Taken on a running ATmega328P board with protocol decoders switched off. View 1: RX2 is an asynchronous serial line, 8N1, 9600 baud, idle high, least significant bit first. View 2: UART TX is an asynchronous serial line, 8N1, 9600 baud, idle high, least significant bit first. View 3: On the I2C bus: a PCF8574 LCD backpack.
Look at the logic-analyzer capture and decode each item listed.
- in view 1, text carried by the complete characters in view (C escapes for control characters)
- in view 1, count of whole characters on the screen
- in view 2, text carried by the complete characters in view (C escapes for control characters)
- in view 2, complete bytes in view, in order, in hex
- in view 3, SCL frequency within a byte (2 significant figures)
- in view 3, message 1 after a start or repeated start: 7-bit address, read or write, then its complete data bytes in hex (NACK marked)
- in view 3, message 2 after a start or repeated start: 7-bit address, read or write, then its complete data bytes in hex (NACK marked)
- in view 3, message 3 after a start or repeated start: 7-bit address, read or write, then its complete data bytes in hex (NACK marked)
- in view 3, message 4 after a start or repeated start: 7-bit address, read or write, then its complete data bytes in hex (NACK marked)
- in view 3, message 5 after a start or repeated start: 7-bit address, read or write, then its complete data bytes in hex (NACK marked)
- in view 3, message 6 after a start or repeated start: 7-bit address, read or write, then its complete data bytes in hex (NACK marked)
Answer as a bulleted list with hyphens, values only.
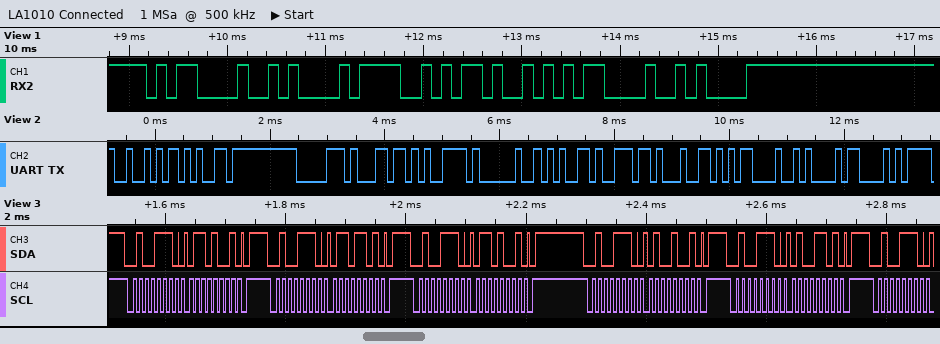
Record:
- "\r\nOK\r\n"
- 6
- "Reply end\r\nC"
- 52 65 70 6C 79 20 65 6E 64 0D 0A 43
- 100 kHz
- 0x27 write: 69
- 0x27 write: 6D
- 0x27 write: 69
- 0x27 write: 49
- 0x27 write: 4D
- 0x27 write
